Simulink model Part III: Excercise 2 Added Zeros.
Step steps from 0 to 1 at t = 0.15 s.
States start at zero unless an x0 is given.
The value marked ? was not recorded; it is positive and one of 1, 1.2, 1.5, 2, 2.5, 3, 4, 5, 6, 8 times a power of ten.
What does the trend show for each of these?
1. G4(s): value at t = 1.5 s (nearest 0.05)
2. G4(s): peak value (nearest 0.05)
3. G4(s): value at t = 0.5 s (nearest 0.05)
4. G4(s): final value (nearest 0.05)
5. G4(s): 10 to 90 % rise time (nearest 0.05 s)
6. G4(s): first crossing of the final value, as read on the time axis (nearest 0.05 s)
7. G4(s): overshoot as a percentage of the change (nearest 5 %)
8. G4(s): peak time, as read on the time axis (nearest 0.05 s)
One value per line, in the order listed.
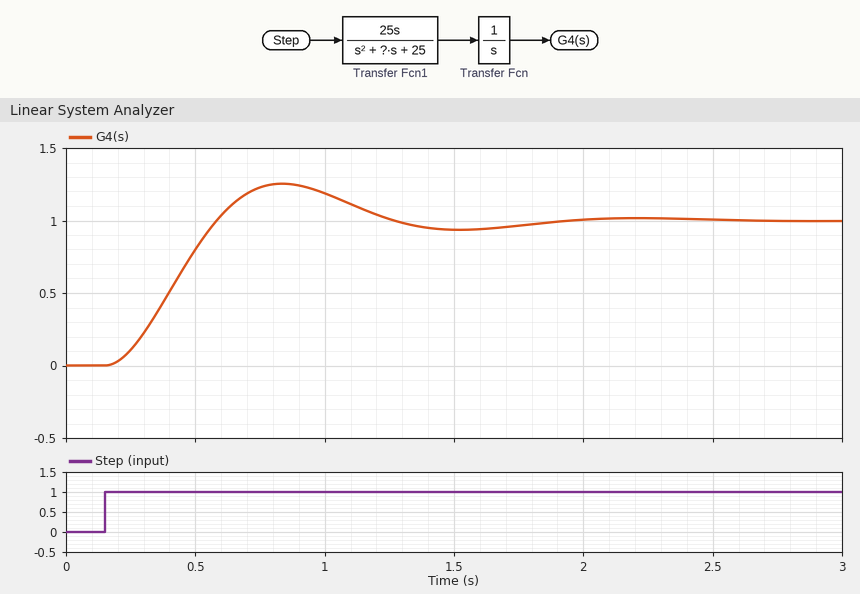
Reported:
0.95
1.25
0.80
1.00
0.30 s
0.60 s
25 %
0.85 s
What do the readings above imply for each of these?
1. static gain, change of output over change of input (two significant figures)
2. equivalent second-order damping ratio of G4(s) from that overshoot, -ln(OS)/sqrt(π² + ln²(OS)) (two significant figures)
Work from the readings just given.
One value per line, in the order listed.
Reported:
1.0
0.40
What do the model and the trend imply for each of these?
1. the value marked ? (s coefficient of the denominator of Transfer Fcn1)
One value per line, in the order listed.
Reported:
4
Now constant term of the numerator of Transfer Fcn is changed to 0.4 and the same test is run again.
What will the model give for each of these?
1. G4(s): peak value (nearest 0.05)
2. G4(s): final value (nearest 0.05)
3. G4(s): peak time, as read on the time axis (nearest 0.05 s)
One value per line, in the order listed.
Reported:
0.50
0.40
0.85 s
